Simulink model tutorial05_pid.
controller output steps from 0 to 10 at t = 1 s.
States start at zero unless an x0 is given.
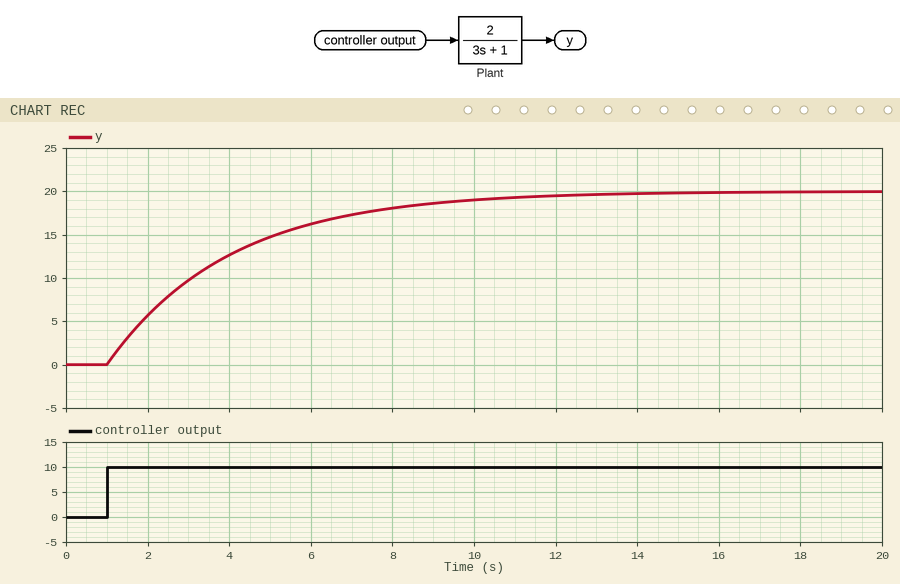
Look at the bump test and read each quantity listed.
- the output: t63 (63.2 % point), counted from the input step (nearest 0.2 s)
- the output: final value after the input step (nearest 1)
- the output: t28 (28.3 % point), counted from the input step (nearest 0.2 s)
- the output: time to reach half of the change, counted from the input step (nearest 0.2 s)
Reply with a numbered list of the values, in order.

1. 3.0 s
2. 20
3. 1.0 s
4. 2.0 s
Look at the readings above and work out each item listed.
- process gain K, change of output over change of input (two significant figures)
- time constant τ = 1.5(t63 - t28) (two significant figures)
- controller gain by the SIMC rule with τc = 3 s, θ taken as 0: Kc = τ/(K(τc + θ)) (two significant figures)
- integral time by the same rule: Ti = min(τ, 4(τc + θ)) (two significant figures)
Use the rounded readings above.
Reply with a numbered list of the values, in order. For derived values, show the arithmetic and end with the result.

1. (20 - 0) / 10 = 2.0
2. 1.5 × (3 - 1) = 3.0 s
3. 3 / (2 × (3 + 0)) = 0.50
4. min(3, 4 × (3 + 0)) = 3.0 s
